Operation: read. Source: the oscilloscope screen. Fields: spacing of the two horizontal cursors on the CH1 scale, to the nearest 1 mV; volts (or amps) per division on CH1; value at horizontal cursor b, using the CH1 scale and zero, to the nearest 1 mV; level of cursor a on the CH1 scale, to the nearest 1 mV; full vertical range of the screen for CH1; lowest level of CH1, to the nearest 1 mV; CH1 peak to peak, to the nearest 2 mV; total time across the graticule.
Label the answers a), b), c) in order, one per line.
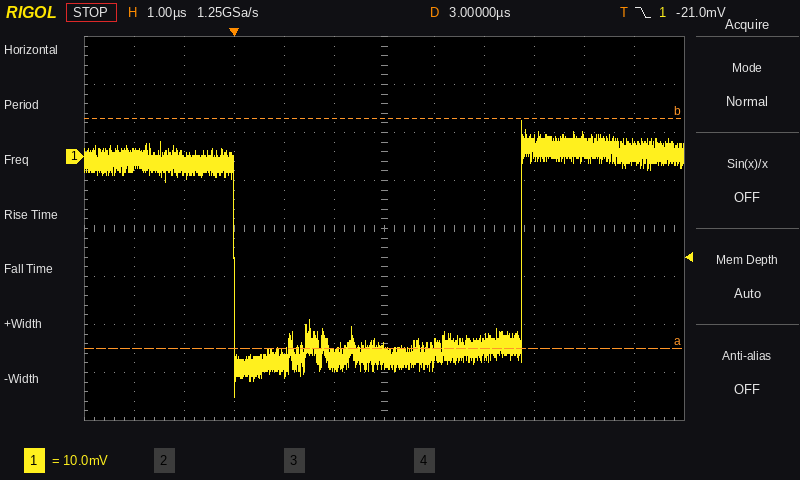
a) 48 mV
b) 10 mV
c) 8 mV
d) -40 mV
e) 80 mV
f) -50 mV
g) 58 mV
h) 12 µs
